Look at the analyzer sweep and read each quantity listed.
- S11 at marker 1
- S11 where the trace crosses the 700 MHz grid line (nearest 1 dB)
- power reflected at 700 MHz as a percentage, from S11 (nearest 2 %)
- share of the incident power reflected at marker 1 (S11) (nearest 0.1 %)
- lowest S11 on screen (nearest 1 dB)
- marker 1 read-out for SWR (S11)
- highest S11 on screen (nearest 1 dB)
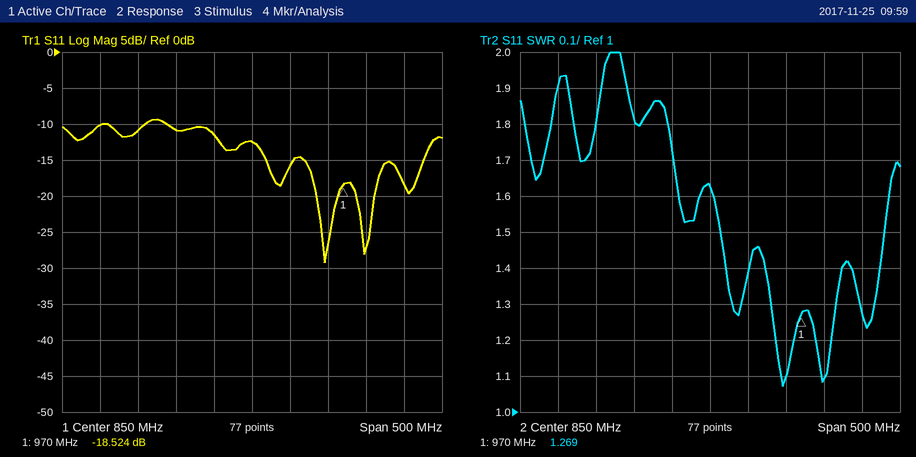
-18.524 dB
-11 dB
8 %
1.4 %
-29 dB
1.269
-9 dB
